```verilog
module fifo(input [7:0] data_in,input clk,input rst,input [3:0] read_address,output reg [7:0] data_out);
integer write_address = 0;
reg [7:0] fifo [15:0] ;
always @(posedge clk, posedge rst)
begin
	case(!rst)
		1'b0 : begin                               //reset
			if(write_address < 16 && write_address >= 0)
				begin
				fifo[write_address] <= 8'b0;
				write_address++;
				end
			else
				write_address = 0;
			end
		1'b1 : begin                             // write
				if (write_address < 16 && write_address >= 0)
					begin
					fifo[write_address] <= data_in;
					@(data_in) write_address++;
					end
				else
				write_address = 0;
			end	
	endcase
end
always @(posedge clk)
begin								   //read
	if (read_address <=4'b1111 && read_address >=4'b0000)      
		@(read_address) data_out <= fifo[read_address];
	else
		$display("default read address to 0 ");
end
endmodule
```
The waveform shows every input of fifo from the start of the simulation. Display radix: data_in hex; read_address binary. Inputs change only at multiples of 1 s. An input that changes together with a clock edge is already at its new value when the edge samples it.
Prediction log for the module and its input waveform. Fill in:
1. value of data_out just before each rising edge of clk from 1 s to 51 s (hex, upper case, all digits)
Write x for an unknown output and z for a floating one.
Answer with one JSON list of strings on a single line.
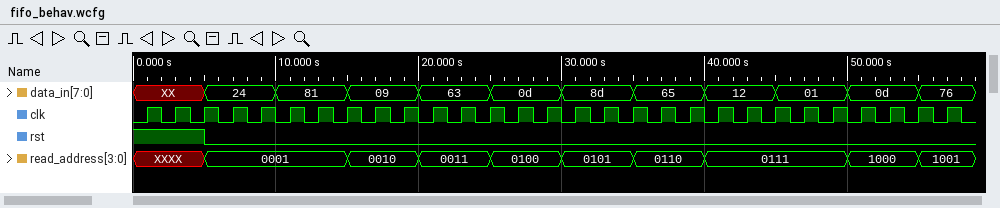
["x, x, x, x, x, x, x, x, 00, 00, 24, 24, 24, 81, 81, 09, 09, 09, 63, 63, 0D, 0D, 0D, 0D, 0D, 8D"]
